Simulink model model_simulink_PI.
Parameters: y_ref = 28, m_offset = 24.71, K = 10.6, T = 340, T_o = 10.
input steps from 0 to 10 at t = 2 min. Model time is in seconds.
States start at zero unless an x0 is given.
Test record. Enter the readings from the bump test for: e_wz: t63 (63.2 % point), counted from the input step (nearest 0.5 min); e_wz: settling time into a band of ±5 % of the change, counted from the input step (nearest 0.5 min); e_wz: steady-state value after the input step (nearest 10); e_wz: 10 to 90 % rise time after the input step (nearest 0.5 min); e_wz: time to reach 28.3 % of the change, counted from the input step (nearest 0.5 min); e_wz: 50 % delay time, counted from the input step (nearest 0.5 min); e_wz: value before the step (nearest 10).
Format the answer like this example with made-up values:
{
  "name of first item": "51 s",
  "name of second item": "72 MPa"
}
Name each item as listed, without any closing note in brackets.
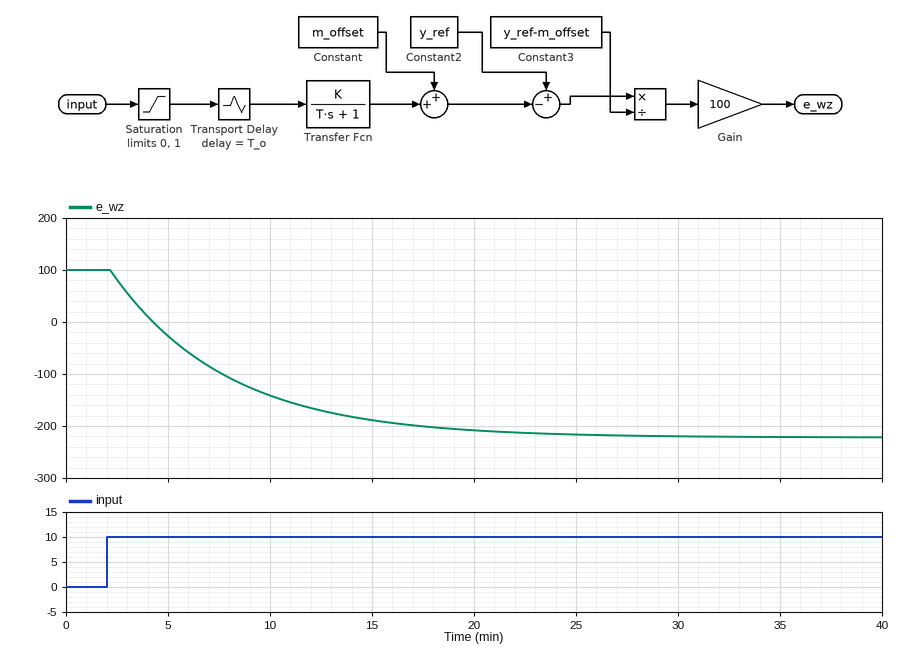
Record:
{
  "e_wz: t63 (63.2 % point), counted from the input step": "6.0 min",
  "e_wz: settling time into a band of ±5 % of the change, counted from the input step": "17.0 min",
  "e_wz: steady-state value after the input step": "-220",
  "e_wz: 10 to 90 % rise time after the input step": "12.5 min",
  "e_wz: time to reach 28.3 % of the change, counted from the input step": "2.0 min",
  "e_wz: 50 % delay time, counted from the input step": "4.0 min",
  "e_wz: value before the step": "100"
}
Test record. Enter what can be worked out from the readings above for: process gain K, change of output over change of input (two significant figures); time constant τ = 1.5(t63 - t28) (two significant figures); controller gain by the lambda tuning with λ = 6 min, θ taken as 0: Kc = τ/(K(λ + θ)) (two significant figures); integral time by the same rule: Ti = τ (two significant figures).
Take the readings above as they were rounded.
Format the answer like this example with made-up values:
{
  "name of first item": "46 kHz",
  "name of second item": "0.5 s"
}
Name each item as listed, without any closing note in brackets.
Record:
{
  "process gain K, change of output over change of input": "-32",
  "time constant τ = 1.5(t63 - t28)": "6.0 min",
  "controller gain by the lambda tuning with λ = 6 min, θ taken as 0: Kc = τ/(K(λ + θ))": "-0.031",
  "integral time by the same rule: Ti = τ": "6.0 min"
}
